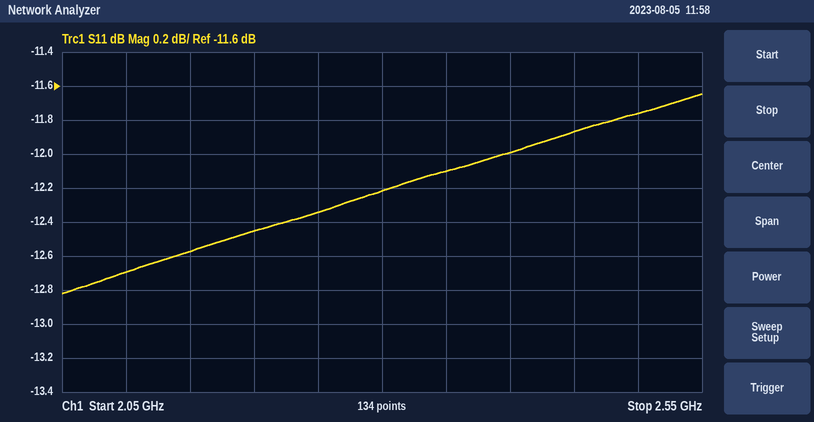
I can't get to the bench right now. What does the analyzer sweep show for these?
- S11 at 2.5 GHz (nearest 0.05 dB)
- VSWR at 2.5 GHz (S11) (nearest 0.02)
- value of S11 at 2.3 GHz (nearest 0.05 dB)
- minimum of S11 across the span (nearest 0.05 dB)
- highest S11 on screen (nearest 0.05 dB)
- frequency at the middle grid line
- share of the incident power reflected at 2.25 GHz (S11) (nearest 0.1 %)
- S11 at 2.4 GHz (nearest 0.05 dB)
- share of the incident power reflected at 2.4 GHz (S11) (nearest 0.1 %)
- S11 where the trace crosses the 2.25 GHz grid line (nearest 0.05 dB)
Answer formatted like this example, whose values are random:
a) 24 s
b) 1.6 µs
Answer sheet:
a) -11.75 dB
b) 1.70
c) -12.20 dB
d) -12.80 dB
e) -11.65 dB
f) 2.3 GHz
g) 5.8 %
h) -12.00 dB
i) 6.3 %
j) -12.35 dB
